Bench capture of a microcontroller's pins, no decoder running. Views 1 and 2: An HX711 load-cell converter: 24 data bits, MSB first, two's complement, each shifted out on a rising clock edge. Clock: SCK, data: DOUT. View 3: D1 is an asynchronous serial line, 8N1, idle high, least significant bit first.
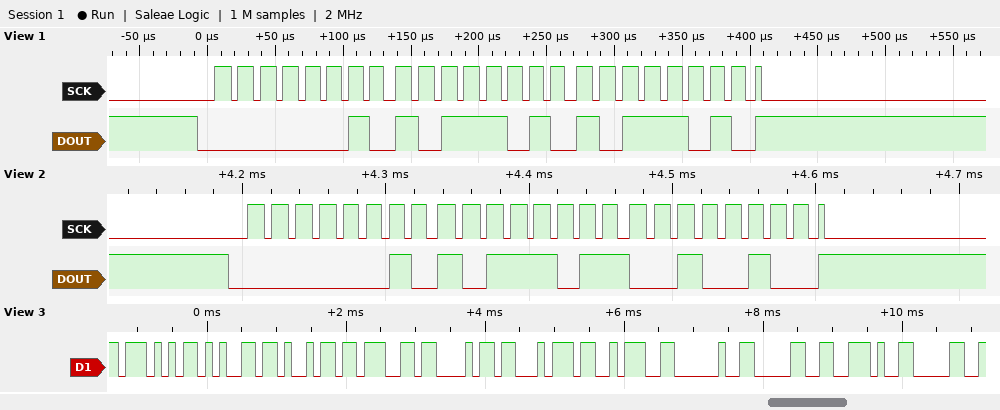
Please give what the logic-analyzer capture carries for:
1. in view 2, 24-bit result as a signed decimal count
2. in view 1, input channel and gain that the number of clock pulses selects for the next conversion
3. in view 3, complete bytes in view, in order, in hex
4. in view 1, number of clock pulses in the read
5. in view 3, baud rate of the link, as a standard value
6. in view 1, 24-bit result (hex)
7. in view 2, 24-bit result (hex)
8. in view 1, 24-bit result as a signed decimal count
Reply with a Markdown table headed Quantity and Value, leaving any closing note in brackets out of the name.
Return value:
| Quantity | Value |
|---|---|
| in view 2, 24-bit result as a signed decimal count | 178980 |
| in view 1, input channel and gain that the number of clock pulses selects for the next conversion | channel A, gain 128 |
| in view 3, complete bytes in view, in order, in hex | 57 65 69 67 68 74 3A 20 30 2E 30 |
| in view 1, number of clock pulses in the read | 25 |
| in view 3, baud rate of the link, as a standard value | 9600 baud |
| in view 1, 24-bit result | 0x02BABA |
| in view 2, 24-bit result | 0x02BB24 |
| in view 1, 24-bit result as a signed decimal count | 178874 |
